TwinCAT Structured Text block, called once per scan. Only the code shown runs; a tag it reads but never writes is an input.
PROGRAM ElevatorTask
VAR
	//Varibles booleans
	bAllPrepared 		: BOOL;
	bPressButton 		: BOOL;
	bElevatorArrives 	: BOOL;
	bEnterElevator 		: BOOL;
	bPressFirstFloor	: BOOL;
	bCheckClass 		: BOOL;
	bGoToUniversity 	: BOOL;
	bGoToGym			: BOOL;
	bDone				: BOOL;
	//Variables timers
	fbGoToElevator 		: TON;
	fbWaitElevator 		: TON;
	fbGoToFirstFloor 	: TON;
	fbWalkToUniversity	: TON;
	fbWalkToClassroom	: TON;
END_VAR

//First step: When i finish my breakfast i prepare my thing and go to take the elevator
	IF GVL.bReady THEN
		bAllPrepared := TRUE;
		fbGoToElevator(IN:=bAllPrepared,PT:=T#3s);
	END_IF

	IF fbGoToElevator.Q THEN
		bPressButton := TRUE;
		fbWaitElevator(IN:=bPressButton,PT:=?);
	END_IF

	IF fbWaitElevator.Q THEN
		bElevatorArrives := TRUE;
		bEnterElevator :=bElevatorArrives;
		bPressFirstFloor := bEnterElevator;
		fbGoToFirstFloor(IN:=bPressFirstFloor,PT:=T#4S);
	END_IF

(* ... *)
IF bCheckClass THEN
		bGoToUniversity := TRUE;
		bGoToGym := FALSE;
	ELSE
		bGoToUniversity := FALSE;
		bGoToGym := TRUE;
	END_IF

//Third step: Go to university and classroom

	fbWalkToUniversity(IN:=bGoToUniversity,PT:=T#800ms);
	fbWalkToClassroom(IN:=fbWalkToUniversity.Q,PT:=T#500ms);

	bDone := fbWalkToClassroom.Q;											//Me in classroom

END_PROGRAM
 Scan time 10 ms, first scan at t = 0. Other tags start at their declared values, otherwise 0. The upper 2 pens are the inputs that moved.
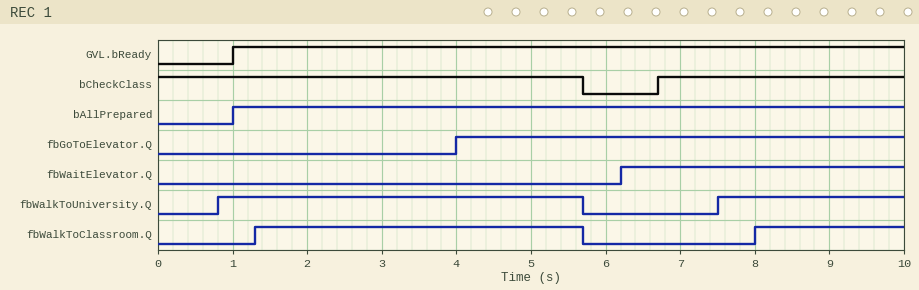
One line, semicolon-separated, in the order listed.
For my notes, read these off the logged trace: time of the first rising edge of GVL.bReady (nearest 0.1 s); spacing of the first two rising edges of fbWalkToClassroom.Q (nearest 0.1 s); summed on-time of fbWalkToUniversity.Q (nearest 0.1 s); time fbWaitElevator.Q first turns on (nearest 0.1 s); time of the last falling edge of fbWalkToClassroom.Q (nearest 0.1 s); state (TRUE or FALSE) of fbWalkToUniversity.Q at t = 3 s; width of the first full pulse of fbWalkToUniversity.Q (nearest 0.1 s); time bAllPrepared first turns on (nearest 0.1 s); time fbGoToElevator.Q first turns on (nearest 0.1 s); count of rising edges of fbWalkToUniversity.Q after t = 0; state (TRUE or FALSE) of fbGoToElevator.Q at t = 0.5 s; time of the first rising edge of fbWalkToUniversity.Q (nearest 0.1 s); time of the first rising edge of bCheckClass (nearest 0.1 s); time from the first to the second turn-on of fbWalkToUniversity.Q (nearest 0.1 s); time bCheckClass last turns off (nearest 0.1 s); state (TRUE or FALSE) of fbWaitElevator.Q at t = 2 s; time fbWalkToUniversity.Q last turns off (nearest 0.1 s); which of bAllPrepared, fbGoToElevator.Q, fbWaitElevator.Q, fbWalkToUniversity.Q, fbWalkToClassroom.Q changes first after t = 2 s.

1.0 s; 6.7 s; 7.4 s; 6.2 s; 5.7 s; TRUE; 4.9 s; 1.0 s; 4.0 s; 2; FALSE; 0.8 s; 6.7 s; 6.7 s; 5.7 s; FALSE; 5.7 s; fbGoToElevator.Q
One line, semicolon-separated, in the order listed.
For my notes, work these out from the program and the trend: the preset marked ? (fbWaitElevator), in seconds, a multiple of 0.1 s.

2.2 s
